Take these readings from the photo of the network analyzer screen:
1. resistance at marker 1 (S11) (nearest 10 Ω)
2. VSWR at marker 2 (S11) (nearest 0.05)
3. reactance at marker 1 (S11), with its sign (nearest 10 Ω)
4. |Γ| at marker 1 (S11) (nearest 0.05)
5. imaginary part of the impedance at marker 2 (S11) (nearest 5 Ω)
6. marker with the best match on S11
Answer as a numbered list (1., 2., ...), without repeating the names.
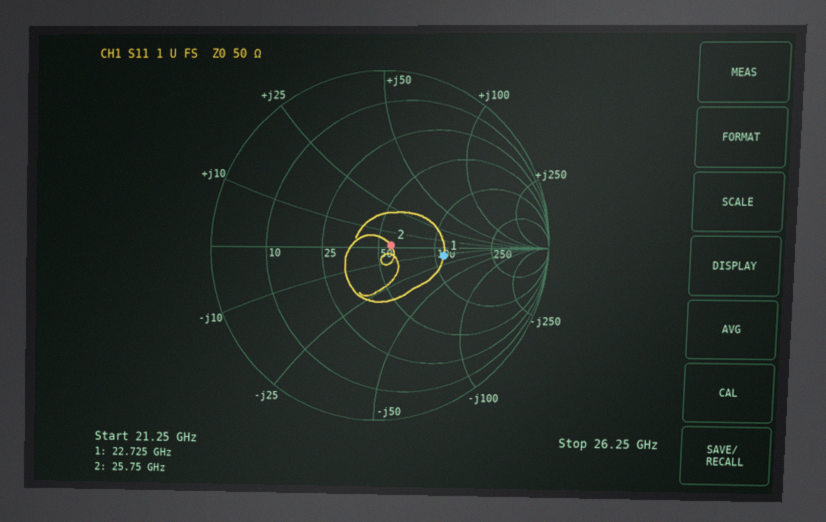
1. 110 Ω
2. 1.15
3. -10 Ω
4. 0.40
5. 0 Ω
6. marker 2
